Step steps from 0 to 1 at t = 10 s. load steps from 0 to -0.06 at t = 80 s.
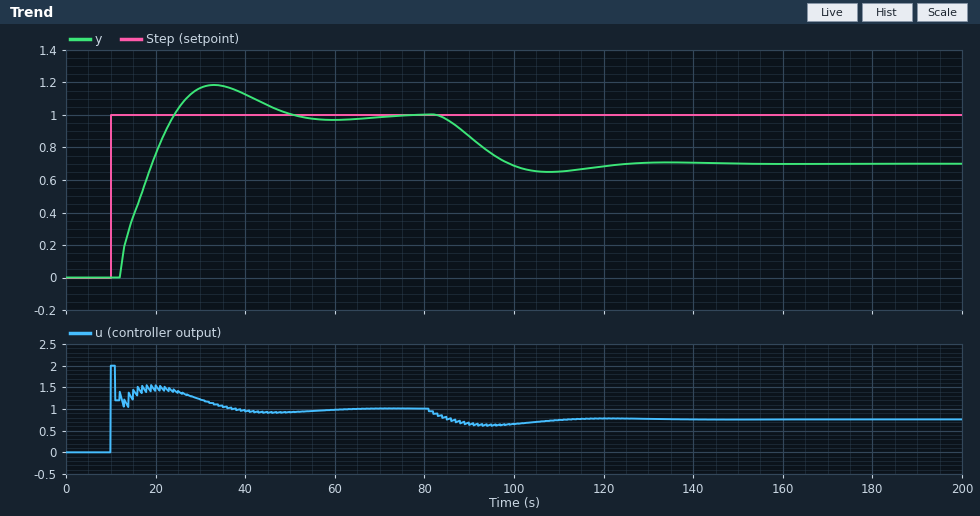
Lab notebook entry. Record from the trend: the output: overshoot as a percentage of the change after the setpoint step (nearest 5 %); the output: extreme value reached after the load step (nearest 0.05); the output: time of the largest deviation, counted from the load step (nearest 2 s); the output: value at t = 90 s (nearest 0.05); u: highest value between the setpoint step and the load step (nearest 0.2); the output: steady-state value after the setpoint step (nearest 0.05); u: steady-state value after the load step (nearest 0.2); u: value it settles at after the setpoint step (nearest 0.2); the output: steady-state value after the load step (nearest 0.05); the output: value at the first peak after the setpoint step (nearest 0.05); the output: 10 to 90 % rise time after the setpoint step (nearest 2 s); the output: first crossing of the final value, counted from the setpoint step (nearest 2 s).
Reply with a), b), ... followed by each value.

a) 20 %
b) 0.65
c) 28 s
d) 0.85
e) 2.0
f) 1.00
g) 0.8
h) 1.0
i) 0.70
j) 1.20
k) 10 s
l) 14 s
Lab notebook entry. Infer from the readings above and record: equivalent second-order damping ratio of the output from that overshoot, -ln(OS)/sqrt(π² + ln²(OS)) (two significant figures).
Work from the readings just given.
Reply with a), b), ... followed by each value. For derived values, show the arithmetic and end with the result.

a) ln(0.2) = -1.609; 1.609 / sqrt(9.870 + 2.590) = 0.46
